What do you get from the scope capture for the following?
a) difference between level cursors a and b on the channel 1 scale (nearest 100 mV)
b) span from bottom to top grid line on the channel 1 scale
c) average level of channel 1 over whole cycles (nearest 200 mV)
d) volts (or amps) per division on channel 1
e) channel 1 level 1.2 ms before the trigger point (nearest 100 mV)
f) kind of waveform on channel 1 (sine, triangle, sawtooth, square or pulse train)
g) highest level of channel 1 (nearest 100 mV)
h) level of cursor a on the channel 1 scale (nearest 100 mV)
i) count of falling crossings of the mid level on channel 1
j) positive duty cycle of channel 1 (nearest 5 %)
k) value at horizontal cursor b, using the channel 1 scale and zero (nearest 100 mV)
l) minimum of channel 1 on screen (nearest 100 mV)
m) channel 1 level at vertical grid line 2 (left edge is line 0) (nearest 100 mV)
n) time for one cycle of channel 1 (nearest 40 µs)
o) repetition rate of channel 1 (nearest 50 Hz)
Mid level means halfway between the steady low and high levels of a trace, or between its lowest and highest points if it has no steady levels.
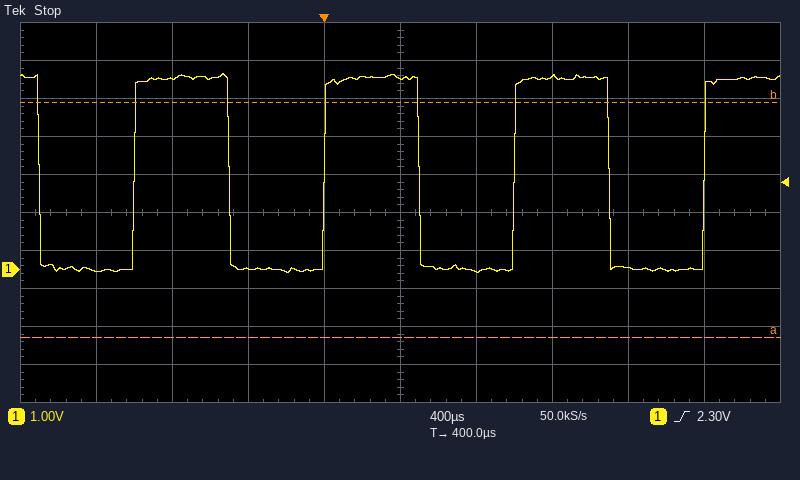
6.2 V
10 V
2.6 V
1 V
0.0 V
square
5.2 V
-1.8 V
4
50 %
4.4 V
-100 mV
5.0 V
1.00 ms
1.00 kHz
